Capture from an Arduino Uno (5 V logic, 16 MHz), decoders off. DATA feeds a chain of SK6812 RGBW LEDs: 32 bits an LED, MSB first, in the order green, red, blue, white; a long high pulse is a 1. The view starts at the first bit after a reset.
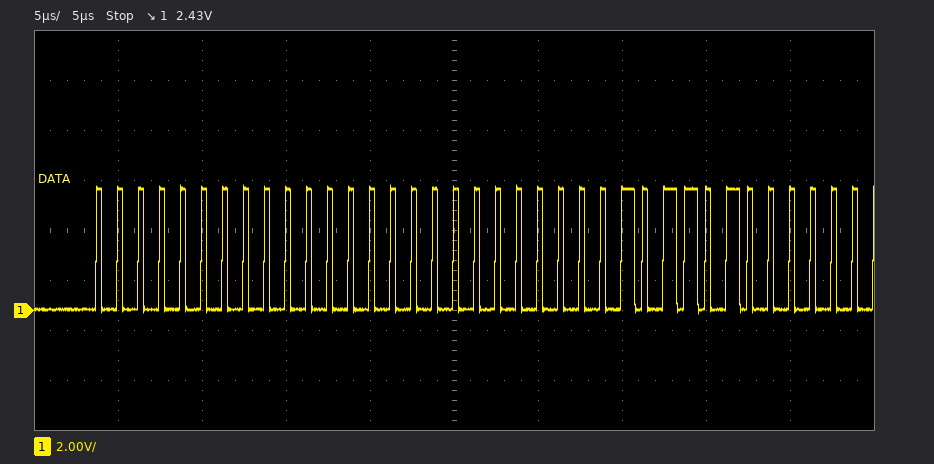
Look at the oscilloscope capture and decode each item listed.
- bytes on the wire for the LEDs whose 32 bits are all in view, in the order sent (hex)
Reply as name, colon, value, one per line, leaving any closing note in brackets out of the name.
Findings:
bytes on the wire for the LEDs whose 32 bits are all in view, in the order sent: 00 00 00 5A
